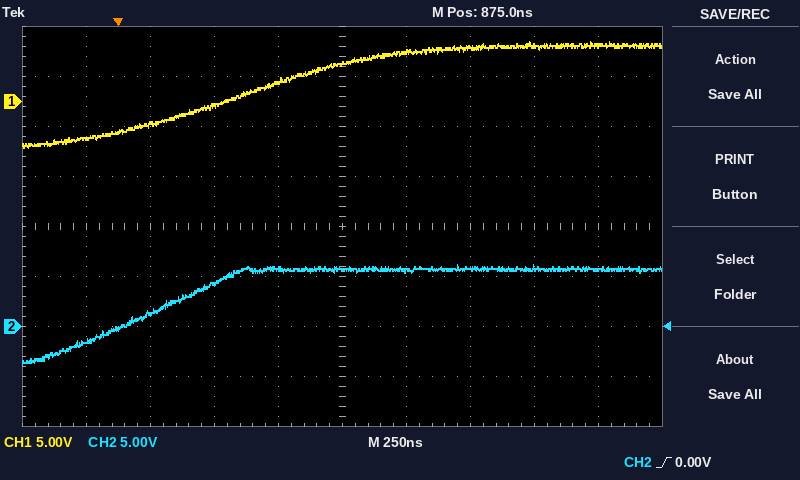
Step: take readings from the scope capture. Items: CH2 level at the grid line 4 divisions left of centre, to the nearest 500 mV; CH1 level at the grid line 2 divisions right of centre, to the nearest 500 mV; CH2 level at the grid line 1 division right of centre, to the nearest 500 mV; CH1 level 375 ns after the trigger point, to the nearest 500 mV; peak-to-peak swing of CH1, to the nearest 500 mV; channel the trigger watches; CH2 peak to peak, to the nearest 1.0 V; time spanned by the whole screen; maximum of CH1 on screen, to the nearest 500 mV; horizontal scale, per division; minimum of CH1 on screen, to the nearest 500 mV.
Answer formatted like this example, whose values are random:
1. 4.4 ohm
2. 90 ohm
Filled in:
1. -1.5 V
2. 5.5 V
3. 5.5 V
4. -500 mV
5. 10.5 V
6. CH2
7. 10.0 V
8. 2.5 µs
9. 6.0 V
10. 250 ns
11. -4.5 V
